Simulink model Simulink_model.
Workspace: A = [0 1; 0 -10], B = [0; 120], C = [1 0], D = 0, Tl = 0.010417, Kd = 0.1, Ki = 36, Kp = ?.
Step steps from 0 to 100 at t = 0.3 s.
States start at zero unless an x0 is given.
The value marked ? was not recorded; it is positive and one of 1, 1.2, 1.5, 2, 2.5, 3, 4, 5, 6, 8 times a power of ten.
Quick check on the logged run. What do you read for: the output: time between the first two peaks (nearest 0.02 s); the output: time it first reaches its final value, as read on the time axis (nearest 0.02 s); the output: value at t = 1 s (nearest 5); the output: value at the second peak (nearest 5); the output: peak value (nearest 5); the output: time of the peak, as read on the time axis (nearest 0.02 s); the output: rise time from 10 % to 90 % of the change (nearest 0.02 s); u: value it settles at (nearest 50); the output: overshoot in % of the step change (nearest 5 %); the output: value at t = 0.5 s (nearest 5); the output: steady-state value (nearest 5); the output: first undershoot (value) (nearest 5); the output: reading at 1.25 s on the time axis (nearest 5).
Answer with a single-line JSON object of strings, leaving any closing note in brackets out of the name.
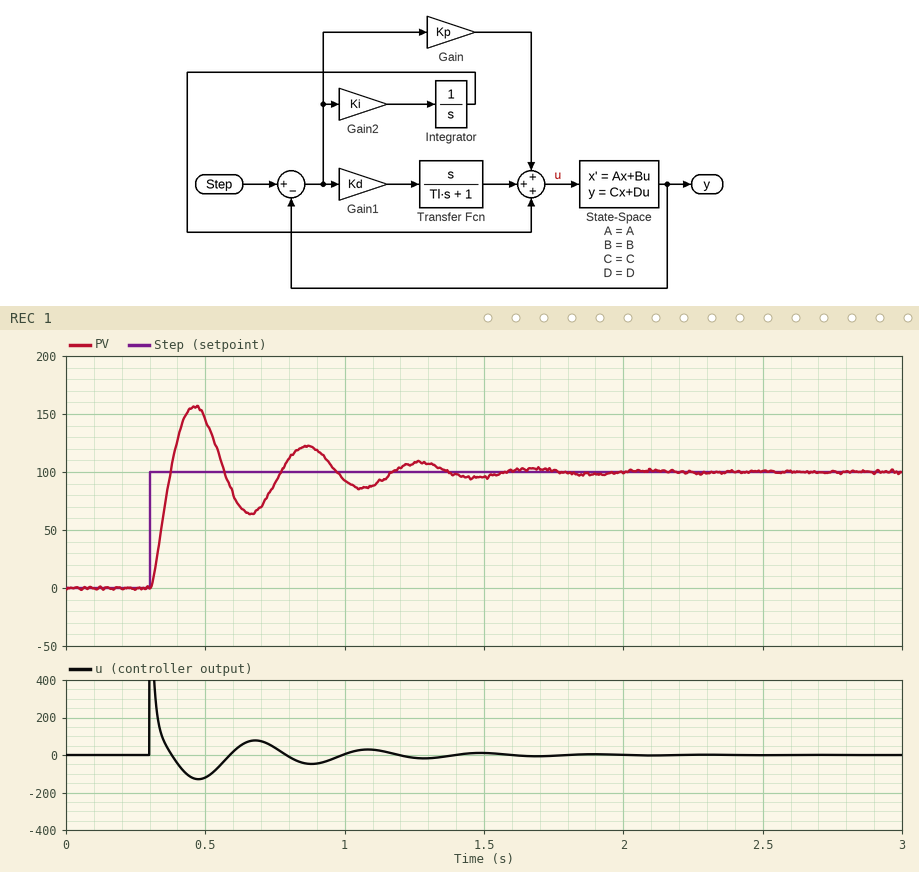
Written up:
{"the output: time between the first two peaks": "0.40 s", "the output: time it first reaches its final value, as read on the time axis": "0.38 s", "the output: value at t = 1 s": "95", "the output: value at the second peak": "120", "the output: peak value": "155", "the output: time of the peak, as read on the time axis": "0.46 s", "the output: rise time from 10 % to 90 % of the change": "0.06 s", "u: value it settles at": "0", "the output: overshoot in % of the step change": "55 %", "the output: value at t = 0.5 s": "145", "the output: steady-state value": "100", "the output: first undershoot (value)": "65", "the output: reading at 1.25 s on the time axis": "110"}
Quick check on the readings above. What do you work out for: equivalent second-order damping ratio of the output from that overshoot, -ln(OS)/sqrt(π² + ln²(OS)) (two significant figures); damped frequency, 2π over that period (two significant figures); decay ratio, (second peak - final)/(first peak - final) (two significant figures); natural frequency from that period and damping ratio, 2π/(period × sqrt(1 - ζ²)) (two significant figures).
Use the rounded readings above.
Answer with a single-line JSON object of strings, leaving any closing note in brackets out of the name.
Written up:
{"equivalent second-order damping ratio of the output from that overshoot, -ln(OS)/sqrt(π² + ln²(OS))": "0.19", "damped frequency, 2π over that period": "16 rad/s", "decay ratio, (second peak - final)/(first peak - final)": "0.36", "natural frequency from that period and damping ratio, 2π/(period × sqrt(1 - ζ²))": "16 rad/s"}
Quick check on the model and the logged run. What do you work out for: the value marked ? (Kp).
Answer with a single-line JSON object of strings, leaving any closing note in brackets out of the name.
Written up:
{"the value marked ?": "2.5"}
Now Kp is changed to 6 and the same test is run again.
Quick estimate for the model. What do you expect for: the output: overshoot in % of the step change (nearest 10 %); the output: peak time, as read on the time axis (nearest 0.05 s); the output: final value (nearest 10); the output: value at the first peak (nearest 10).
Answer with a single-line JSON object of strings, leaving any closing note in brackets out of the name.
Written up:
{"the output: overshoot in % of the step change": "50 %", "the output: peak time, as read on the time axis": "0.40 s", "the output: final value": "100", "the output: value at the first peak": "150"}
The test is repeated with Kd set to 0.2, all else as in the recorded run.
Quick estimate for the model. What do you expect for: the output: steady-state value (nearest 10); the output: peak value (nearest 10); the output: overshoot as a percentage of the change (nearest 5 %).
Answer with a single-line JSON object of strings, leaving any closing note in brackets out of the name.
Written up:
{"the output: steady-state value": "100", "the output: peak value": "130", "the output: overshoot as a percentage of the change": "30 %"}
